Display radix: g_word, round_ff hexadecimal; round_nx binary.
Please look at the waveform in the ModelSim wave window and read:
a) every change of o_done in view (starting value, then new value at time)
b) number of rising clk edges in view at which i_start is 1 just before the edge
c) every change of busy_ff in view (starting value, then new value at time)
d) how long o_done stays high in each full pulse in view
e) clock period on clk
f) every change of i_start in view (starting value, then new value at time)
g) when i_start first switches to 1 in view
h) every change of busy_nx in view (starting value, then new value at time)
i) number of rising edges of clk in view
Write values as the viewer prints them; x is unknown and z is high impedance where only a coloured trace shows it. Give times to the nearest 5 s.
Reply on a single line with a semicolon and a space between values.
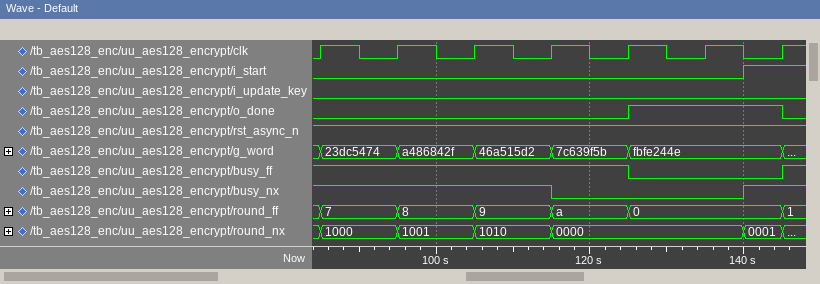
0, 1 at 125 s, 0 at 145 s; 1; 1, 0 at 125 s, 1 at 145 s; 20 s; 10 s; 0, 1 at 140 s; 140 s; 1, 0 at 115 s, 1 at 140 s; 7
